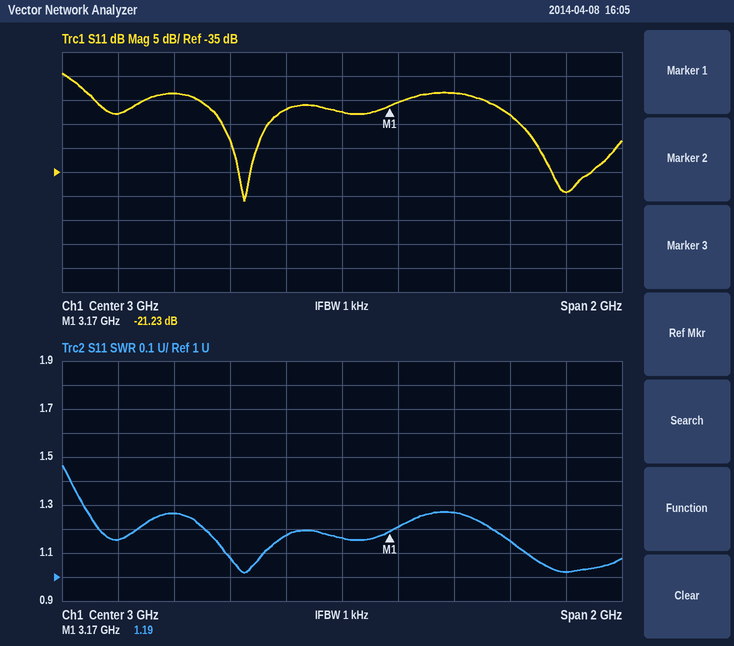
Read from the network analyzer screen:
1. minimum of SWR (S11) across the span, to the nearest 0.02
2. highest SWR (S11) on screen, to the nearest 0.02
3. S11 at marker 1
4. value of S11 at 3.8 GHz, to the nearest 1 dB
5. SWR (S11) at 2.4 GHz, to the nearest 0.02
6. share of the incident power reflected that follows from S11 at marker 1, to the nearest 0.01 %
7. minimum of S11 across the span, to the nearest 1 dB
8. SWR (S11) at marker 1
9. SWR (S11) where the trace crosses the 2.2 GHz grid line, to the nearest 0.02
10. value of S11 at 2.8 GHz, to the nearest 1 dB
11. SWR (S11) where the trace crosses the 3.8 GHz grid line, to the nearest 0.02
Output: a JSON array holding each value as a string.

["1.02", "1.46", "-21.23 dB", "-39 dB", "1.26", "0.75 %", "-41 dB", "1.19", "1.16", "-22 dB", "1.02"]
